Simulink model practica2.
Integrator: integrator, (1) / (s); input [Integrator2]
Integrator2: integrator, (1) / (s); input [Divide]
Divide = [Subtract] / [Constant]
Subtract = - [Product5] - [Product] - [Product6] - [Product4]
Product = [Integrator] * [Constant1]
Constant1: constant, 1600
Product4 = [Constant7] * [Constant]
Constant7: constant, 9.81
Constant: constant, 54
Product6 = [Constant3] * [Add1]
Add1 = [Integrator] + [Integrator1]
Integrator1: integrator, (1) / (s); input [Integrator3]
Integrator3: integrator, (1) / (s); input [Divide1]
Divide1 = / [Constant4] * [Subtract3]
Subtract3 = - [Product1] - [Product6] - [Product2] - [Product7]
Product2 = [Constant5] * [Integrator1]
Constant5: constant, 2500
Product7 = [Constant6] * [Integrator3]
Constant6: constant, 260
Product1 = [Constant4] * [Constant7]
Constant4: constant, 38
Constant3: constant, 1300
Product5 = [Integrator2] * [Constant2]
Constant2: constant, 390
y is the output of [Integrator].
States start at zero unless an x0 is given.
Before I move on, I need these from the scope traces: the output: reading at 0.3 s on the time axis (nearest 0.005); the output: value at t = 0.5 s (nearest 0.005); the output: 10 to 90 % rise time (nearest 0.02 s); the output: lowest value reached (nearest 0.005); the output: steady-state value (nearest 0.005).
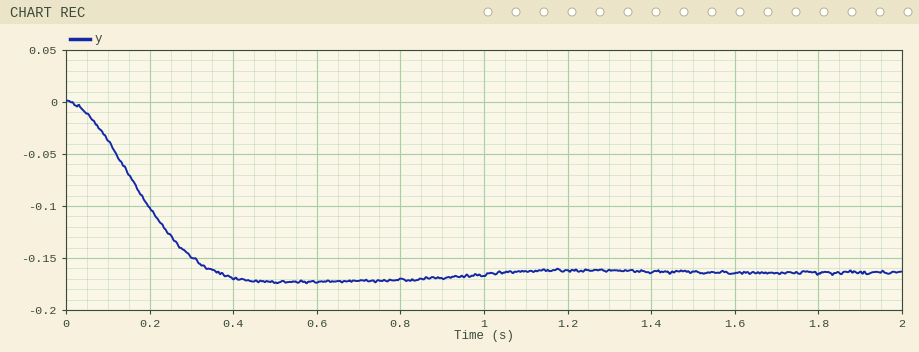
-0.150
-0.175
0.24 s
-0.175
-0.165
